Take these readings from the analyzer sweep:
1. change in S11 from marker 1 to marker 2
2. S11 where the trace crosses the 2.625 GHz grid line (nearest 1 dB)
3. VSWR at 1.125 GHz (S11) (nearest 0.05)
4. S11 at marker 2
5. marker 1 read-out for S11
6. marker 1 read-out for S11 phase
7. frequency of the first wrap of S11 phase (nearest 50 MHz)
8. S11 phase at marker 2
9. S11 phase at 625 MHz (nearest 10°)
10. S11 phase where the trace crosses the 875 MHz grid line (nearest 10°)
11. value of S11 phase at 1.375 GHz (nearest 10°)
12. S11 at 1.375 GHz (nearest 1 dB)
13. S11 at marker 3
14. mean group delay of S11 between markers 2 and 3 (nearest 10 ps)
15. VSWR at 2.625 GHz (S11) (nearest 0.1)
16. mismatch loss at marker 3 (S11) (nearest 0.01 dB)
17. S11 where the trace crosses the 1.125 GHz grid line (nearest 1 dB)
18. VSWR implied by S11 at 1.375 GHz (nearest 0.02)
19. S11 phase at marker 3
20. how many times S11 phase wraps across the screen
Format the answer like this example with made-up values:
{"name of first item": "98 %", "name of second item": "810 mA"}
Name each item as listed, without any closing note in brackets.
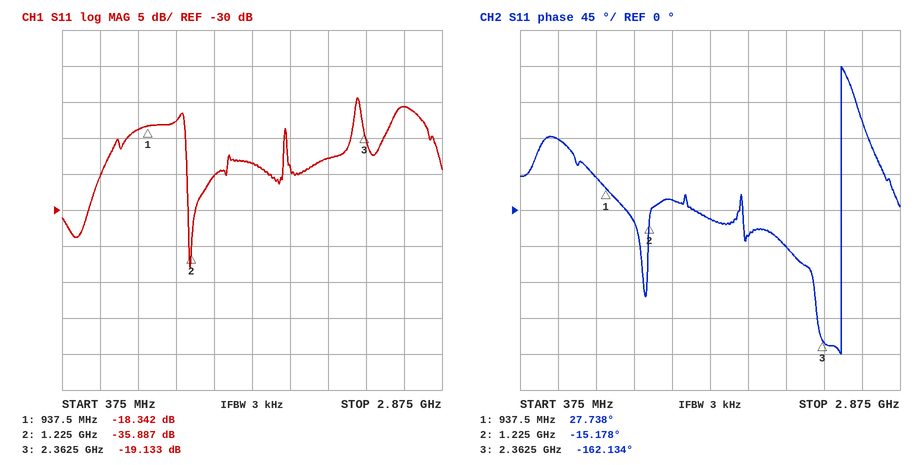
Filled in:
{"change in S11 from marker 1 to marker 2": "-17.545 dB", "S11 where the trace crosses the 2.625 GHz grid line": "-16 dB", "VSWR at 1.125 GHz (S11)": "1.30", "S11 at marker 2": "-35.887 dB", "marker 1 read-out for S11": "-18.342 dB", "marker 1 read-out for S11 phase": "27.738°", "frequency of the first wrap of S11 phase": "2.50 GHz", "S11 phase at marker 2": "-15.178°", "S11 phase at 625 MHz": "90°", "S11 phase where the trace crosses the 875 MHz grid line": "40°", "value of S11 phase at 1.375 GHz": "10°", "S11 at 1.375 GHz": "-25 dB", "S11 at marker 3": "-19.133 dB", "mean group delay of S11 between markers 2 and 3": "360 ps", "VSWR at 2.625 GHz (S11)": "1.4", "mismatch loss at marker 3 (S11)": "0.05 dB", "S11 where the trace crosses the 1.125 GHz grid line": "-18 dB", "VSWR implied by S11 at 1.375 GHz": "1.12", "S11 phase at marker 3": "-162.134°", "how many times S11 phase wraps across the screen": "1"}
